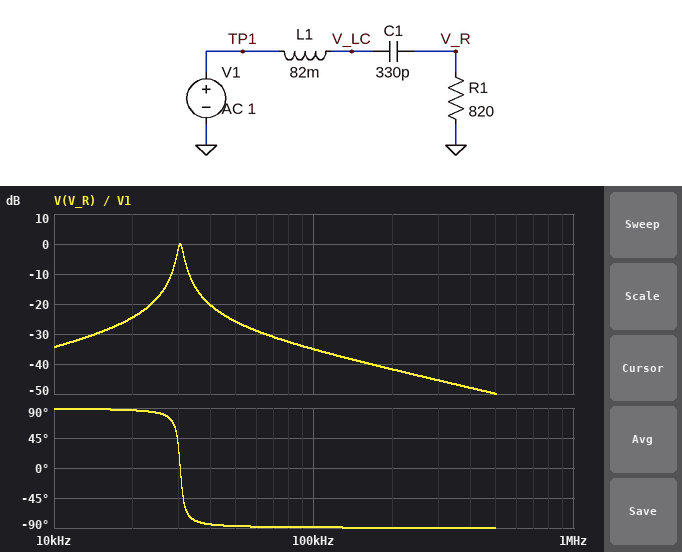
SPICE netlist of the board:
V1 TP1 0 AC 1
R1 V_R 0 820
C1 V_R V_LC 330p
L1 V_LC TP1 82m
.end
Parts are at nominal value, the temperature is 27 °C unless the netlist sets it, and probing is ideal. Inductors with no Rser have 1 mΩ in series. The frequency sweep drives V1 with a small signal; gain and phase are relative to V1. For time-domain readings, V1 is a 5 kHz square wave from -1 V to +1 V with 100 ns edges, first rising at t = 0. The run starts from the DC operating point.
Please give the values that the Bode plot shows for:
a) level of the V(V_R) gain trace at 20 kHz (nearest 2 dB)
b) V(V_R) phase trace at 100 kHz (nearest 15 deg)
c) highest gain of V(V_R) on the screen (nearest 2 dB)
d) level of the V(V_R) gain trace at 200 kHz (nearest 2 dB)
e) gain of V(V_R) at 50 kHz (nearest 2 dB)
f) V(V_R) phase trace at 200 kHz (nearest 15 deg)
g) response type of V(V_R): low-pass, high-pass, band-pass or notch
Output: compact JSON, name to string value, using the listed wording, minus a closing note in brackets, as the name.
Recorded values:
{"level of the V(V_R) gain trace at 20 kHz": "-24 dB", "V(V_R) phase trace at 100 kHz": "-90 deg", "highest gain of V(V_R) on the screen": "0 dB", "level of the V(V_R) gain trace at 200 kHz": "-42 dB", "gain of V(V_R) at 50 kHz": "-26 dB", "V(V_R) phase trace at 200 kHz": "-90 deg", "response type of V(V_R): low-pass, high-pass, band-pass or notch": "band-pass"}
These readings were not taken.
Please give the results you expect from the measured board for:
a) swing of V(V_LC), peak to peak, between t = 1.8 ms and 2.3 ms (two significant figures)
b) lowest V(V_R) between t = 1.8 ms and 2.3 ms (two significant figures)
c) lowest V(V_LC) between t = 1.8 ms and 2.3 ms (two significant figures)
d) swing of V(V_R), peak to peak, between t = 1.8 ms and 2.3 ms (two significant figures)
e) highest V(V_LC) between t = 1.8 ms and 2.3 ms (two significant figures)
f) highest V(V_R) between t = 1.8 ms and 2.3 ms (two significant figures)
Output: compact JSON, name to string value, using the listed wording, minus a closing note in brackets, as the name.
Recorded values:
{"swing of V(V_LC), peak to peak, between t = 1.8 ms and 2.3 ms": "4.3 V", "lowest V(V_R) between t = 1.8 ms and 2.3 ms": "-63 mV", "lowest V(V_LC) between t = 1.8 ms and 2.3 ms": "-2.2 V", "swing of V(V_R), peak to peak, between t = 1.8 ms and 2.3 ms": "130 mV", "highest V(V_LC) between t = 1.8 ms and 2.3 ms": "2.2 V", "highest V(V_R) between t = 1.8 ms and 2.3 ms": "63 mV"}
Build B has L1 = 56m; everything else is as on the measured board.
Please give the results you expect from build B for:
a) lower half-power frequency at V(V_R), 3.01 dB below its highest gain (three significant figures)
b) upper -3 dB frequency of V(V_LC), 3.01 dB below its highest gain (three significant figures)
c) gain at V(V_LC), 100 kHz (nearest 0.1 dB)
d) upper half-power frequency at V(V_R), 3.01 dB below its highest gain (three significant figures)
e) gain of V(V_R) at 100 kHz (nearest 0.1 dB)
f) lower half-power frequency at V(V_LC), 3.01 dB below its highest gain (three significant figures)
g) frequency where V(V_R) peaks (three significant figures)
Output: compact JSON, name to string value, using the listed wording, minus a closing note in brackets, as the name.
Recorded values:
{"lower half-power frequency at V(V_R), 3.01 dB below its highest gain": "35.9 kHz", "upper -3 dB frequency of V(V_LC), 3.01 dB below its highest gain": "38.1 kHz", "gain at V(V_LC), 100 kHz": "-15.9 dB", "upper half-power frequency at V(V_R), 3.01 dB below its highest gain": "38.2 kHz", "gain of V(V_R) at 100 kHz": "-31.4 dB", "lower half-power frequency at V(V_LC), 3.01 dB below its highest gain": "35.8 kHz", "frequency where V(V_R) peaks": "37.0 kHz"}
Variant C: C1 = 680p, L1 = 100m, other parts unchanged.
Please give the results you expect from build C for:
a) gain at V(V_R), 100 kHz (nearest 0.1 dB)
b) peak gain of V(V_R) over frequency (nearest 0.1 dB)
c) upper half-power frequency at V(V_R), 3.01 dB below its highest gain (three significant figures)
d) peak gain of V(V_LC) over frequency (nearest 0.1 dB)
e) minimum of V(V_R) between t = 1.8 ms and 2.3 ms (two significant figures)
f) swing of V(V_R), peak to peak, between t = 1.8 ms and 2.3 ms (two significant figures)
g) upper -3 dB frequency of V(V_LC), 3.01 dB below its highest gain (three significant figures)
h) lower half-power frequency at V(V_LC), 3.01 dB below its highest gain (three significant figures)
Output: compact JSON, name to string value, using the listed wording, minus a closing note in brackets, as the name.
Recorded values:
{"gain at V(V_R), 100 kHz": "-37.4 dB", "peak gain of V(V_R) over frequency": "0 dB", "upper half-power frequency at V(V_R), 3.01 dB below its highest gain": "20.0 kHz", "peak gain of V(V_LC) over frequency": "23.4 dB", "minimum of V(V_R) between t = 1.8 ms and 2.3 ms": "-80 mV", "swing of V(V_R), peak to peak, between t = 1.8 ms and 2.3 ms": "160 mV", "upper -3 dB frequency of V(V_LC), 3.01 dB below its highest gain": "19.9 kHz", "lower half-power frequency at V(V_LC), 3.01 dB below its highest gain": "18.6 kHz"}
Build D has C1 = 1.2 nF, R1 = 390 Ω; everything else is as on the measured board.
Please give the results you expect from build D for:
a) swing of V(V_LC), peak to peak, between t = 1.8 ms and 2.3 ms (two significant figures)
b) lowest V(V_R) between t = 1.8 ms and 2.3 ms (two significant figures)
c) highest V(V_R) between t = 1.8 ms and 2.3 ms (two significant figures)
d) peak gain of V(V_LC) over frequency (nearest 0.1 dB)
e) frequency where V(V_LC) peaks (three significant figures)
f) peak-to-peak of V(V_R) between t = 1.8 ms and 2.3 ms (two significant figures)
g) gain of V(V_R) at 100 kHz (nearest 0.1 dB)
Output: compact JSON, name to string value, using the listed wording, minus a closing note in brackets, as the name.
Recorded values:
{"swing of V(V_LC), peak to peak, between t = 1.8 ms and 2.3 ms": "8.3 V", "lowest V(V_R) between t = 1.8 ms and 2.3 ms": "-150 mV", "highest V(V_R) between t = 1.8 ms and 2.3 ms": "150 mV", "peak gain of V(V_LC) over frequency": "26.5 dB", "frequency where V(V_LC) peaks": "16.0 kHz", "peak-to-peak of V(V_R) between t = 1.8 ms and 2.3 ms": "310 mV", "gain of V(V_R) at 100 kHz": "-42.2 dB"}
